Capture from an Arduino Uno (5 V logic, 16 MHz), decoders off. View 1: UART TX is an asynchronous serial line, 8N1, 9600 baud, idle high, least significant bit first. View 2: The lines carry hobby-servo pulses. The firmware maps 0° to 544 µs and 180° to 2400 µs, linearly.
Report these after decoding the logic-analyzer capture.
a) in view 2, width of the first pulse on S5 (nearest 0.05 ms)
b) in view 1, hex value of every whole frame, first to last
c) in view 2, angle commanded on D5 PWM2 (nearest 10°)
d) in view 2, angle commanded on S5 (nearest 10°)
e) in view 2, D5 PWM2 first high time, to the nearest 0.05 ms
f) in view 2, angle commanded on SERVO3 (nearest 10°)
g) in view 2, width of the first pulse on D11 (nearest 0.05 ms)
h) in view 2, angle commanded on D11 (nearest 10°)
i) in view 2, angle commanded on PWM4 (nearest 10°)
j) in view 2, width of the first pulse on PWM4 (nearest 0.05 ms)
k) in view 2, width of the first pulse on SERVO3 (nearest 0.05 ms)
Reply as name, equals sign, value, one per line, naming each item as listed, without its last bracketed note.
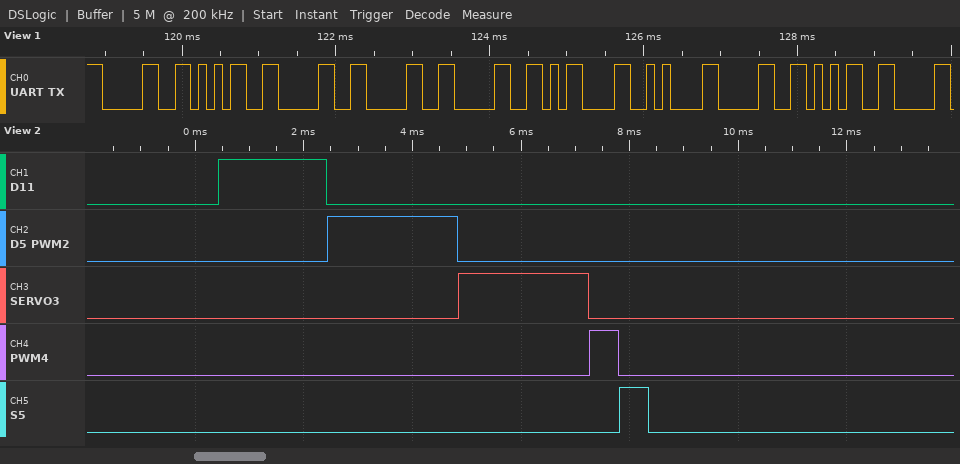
in view 2, width of the first pulse on S5 = 0.55 ms
in view 1, hex value of every whole frame, first to last = 30 35 30 30 30 0D 0A 30 35
in view 2, angle commanded on D5 PWM2 = 180°
in view 2, angle commanded on S5 = 0°
in view 2, D5 PWM2 first high time, to the nearest 0.05 ms = 2.40 ms
in view 2, angle commanded on SERVO3 = 180°
in view 2, width of the first pulse on D11 = 2.00 ms
in view 2, angle commanded on D11 = 140°
in view 2, angle commanded on PWM4 = 0°
in view 2, width of the first pulse on PWM4 = 0.55 ms
in view 2, width of the first pulse on SERVO3 = 2.40 ms
